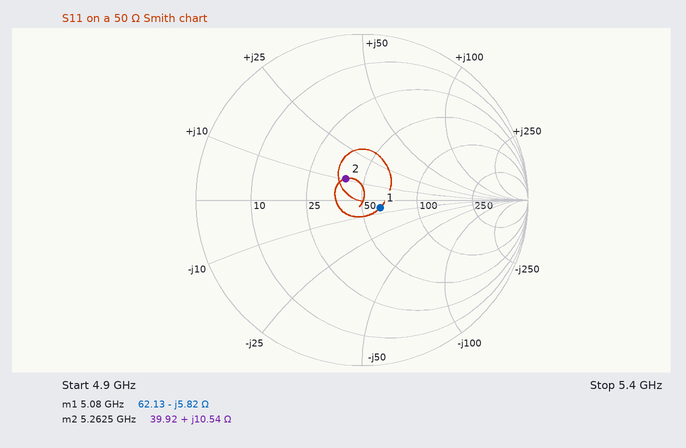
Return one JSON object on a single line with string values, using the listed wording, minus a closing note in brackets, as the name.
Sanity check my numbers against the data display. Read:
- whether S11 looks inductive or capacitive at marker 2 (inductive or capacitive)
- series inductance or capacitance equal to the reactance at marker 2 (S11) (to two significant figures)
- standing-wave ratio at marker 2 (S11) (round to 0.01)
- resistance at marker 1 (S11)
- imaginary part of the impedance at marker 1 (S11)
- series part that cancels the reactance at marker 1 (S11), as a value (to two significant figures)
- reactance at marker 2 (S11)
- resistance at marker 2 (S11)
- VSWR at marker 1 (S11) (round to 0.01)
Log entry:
{"whether S11 looks inductive or capacitive at marker 2": "inductive", "series inductance or capacitance equal to the reactance at marker 2 (S11)": "320 pH", "standing-wave ratio at marker 2 (S11)": "1.38", "resistance at marker 1": "62.13 Ω", "imaginary part of the impedance at marker 1": "-5.82 Ω", "series part that cancels the reactance at marker 1 (S11), as a value": "180 pH", "reactance at marker 2": "+10.54 Ω", "resistance at marker 2": "39.92 Ω", "VSWR at marker 1 (S11)": "1.27"}
